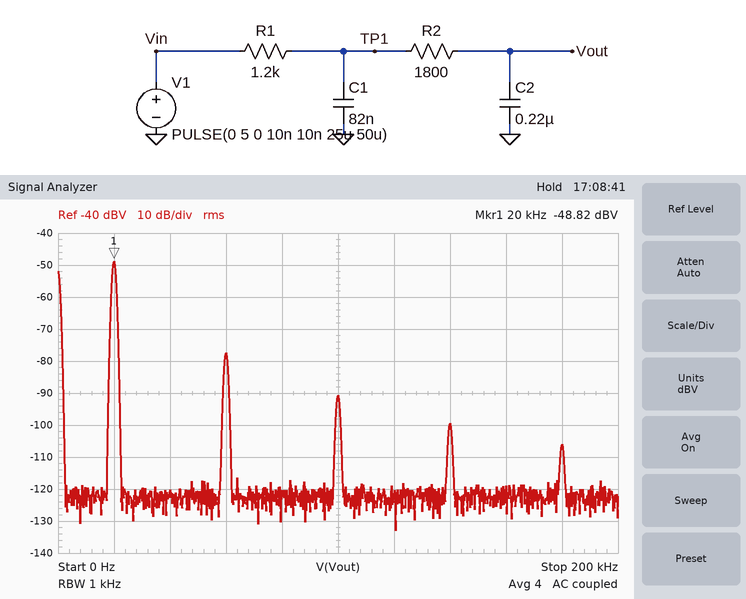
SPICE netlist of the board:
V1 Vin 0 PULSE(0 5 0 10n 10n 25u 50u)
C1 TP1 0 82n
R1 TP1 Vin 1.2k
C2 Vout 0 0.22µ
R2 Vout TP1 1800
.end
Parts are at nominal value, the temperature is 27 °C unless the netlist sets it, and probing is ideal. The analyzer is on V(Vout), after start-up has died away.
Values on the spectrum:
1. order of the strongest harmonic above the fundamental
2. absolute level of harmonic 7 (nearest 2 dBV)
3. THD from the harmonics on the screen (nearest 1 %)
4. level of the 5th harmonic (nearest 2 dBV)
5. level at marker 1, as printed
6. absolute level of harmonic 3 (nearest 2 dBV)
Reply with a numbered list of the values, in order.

1. 3
2. -100 dBV
3. 4 %
4. -90 dBV
5. -48.82 dBV
6. -78 dBV
